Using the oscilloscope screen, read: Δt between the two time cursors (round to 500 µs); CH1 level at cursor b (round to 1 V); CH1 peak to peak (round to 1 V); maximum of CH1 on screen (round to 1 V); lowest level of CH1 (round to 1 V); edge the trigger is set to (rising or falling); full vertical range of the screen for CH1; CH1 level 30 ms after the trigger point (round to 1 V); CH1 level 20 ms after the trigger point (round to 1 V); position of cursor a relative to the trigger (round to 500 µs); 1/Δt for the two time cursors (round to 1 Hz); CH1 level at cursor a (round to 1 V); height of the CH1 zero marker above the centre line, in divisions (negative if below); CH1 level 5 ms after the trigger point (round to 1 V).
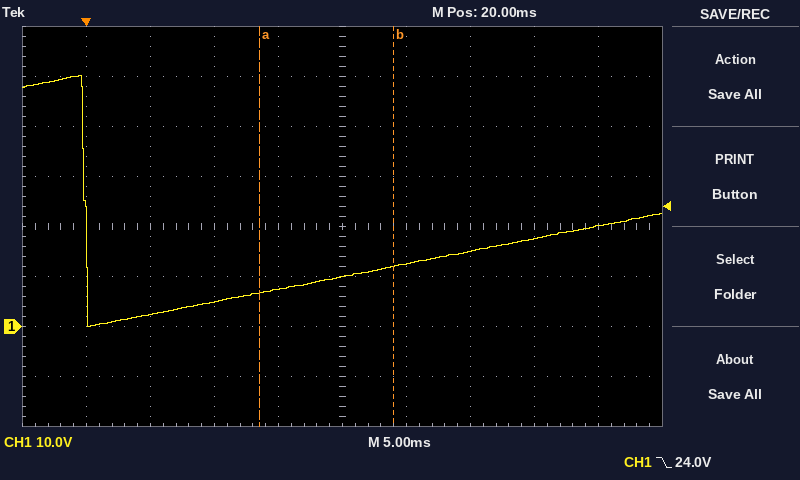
10.5 ms
12 V
50 V
50 V
0 V
falling
80 V
15 V
10 V
+13.5 ms
95 Hz
7 V
-2.0 div
2 V
